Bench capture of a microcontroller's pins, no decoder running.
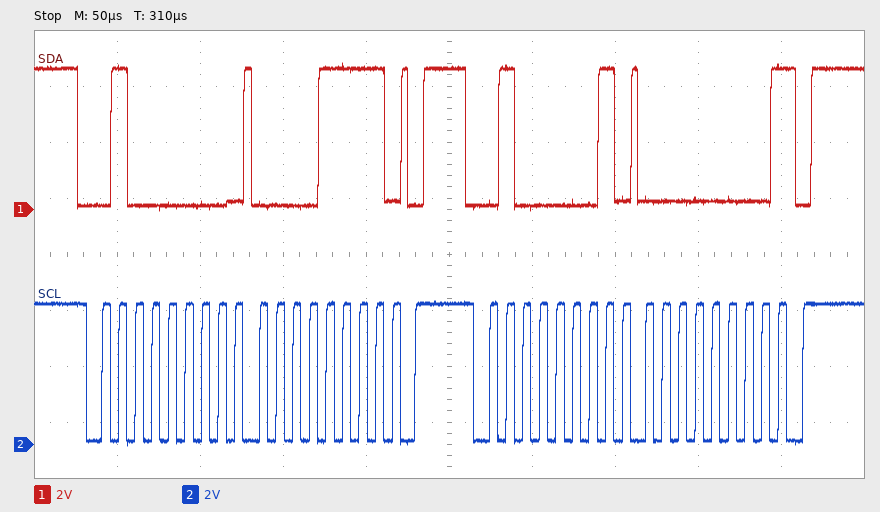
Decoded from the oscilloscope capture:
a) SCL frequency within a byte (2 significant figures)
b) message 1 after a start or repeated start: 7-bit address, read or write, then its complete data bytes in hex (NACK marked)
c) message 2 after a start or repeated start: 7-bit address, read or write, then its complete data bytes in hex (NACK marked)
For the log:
100 kHz
0x20 write: 0F
0x20 read: 00 NACK
